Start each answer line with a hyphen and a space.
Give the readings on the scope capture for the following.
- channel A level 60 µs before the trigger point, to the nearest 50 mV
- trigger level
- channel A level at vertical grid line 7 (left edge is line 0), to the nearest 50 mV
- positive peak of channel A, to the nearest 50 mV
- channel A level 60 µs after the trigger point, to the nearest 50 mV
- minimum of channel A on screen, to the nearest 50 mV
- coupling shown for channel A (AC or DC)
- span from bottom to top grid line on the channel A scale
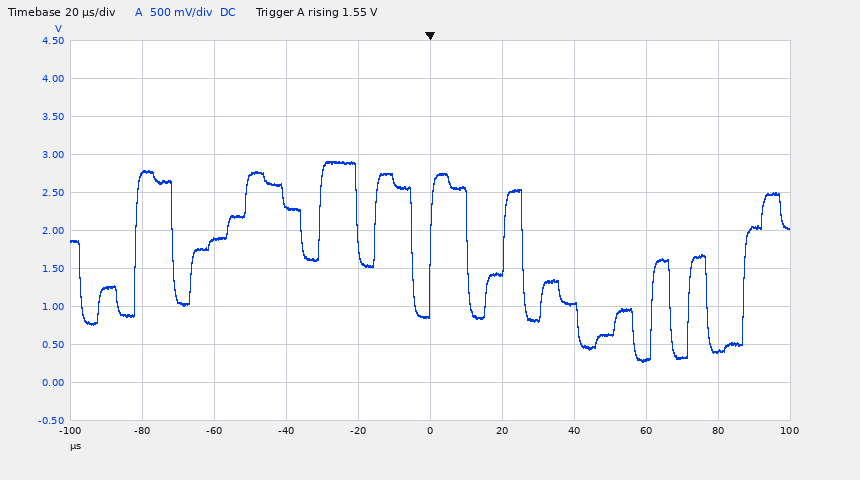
- 1.90 V
- 1.55 V
- 1.00 V
- 2.90 V
- 300 mV
- 300 mV
- DC
- 5 V
